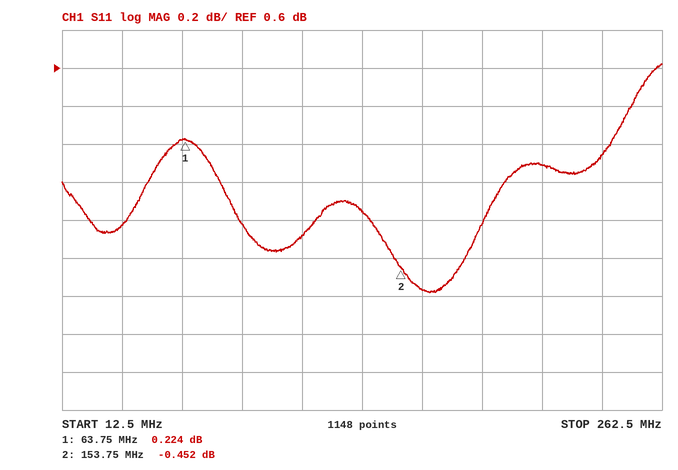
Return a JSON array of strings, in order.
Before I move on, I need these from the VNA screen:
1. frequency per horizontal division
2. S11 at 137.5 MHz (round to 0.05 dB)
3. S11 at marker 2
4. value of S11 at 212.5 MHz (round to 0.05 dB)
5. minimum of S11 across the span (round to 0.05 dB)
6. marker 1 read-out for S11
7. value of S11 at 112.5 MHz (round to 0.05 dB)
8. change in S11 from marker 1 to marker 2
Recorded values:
["25 MHz", "-0.15 dB", "-0.452 dB", "0.10 dB", "-0.60 dB", "0.224 dB", "-0.30 dB", "-0.676 dB"]
